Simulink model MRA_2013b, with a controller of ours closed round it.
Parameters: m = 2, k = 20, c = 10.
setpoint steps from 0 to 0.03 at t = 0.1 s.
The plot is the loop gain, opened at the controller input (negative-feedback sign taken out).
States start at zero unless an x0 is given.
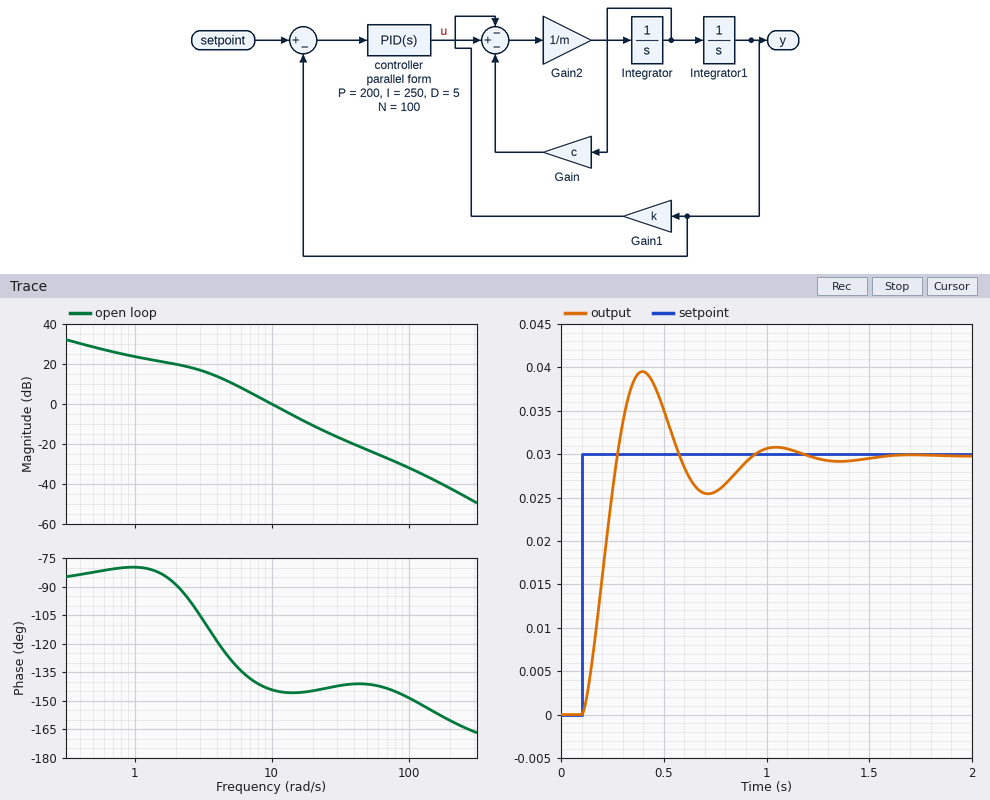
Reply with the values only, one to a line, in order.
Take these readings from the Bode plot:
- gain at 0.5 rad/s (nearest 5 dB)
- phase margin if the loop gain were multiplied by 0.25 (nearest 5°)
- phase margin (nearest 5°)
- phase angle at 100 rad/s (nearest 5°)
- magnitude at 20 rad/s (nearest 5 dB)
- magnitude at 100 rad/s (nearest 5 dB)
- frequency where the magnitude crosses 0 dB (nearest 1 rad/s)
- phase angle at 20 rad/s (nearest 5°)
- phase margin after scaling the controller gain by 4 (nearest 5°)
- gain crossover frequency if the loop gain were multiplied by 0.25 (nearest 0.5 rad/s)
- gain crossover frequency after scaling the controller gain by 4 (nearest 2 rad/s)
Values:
30 dB
55°
35°
-150°
-10 dB
-30 dB
10 rad/s
-145°
35°
4.5 rad/s
22 rad/s
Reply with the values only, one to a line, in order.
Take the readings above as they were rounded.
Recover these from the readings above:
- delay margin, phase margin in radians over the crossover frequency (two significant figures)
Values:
0.061 s
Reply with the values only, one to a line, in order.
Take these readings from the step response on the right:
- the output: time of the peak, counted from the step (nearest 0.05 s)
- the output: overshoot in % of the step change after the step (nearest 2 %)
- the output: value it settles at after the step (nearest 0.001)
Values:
0.30 s
32 %
0.030
